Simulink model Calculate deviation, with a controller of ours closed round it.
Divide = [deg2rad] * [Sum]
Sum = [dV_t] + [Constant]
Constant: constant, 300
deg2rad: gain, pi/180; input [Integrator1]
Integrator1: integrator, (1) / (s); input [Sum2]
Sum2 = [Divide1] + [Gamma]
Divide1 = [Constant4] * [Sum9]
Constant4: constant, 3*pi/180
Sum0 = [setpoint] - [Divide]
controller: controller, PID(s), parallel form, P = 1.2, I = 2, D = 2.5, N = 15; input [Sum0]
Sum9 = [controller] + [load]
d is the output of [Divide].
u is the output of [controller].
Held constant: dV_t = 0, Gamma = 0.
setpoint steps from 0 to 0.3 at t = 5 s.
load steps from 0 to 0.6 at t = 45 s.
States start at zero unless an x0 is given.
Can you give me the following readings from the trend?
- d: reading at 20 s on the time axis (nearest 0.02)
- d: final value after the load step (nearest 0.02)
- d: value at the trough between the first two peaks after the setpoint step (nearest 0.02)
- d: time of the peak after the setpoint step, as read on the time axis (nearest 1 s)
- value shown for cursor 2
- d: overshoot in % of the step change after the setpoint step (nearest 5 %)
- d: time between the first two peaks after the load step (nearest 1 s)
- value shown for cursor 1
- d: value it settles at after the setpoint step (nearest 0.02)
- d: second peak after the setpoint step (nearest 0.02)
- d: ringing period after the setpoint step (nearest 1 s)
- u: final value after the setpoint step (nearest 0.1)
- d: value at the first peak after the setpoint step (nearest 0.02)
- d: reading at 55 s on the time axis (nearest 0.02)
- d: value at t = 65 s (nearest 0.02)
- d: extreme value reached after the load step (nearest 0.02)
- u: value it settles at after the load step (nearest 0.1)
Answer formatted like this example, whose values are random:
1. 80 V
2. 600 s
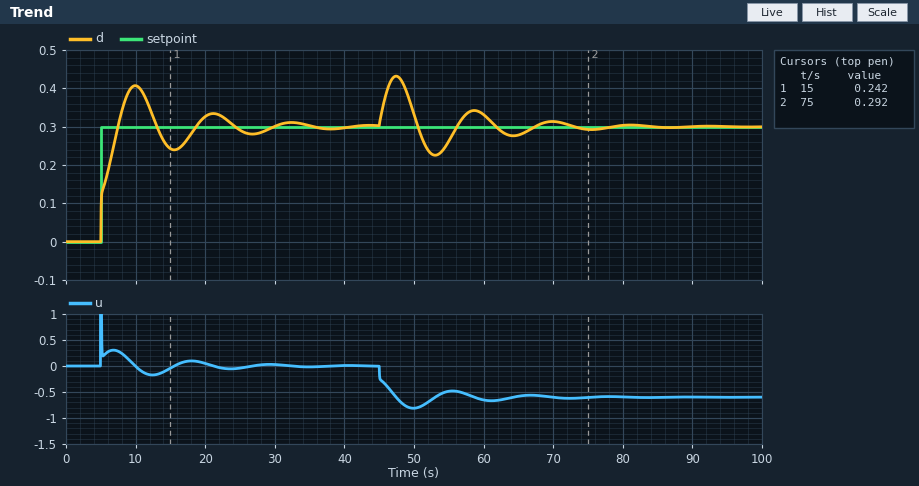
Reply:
1. 0.32
2. 0.30
3. 0.24
4. 10 s
5. 0.292
6. 35 %
7. 11 s
8. 0.242
9. 0.30
10. 0.34
11. 11 s
12. 0.0
13. 0.40
14. 0.26
15. 0.28
16. 0.44
17. -0.6
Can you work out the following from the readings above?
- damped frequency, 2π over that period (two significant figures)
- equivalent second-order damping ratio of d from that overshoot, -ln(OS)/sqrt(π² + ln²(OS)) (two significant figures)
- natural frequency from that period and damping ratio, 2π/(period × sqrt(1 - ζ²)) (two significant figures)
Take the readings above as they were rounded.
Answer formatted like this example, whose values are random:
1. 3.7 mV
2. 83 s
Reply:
1. 0.57 rad/s
2. 0.32
3. 0.60 rad/s
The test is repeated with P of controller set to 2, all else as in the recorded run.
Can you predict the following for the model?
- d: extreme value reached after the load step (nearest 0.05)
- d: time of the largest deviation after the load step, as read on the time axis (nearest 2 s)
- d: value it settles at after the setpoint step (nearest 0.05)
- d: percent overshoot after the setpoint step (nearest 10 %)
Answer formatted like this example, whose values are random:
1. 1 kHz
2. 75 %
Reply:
1. 0.40
2. 48 s
3. 0.30
4. 30 %
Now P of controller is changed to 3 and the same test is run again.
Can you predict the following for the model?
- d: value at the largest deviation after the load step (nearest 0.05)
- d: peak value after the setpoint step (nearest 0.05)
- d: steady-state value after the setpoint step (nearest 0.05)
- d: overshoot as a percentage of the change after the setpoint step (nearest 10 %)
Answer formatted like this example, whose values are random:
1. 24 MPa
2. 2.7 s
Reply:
1. 0.40
2. 0.35
3. 0.30
4. 20 %
